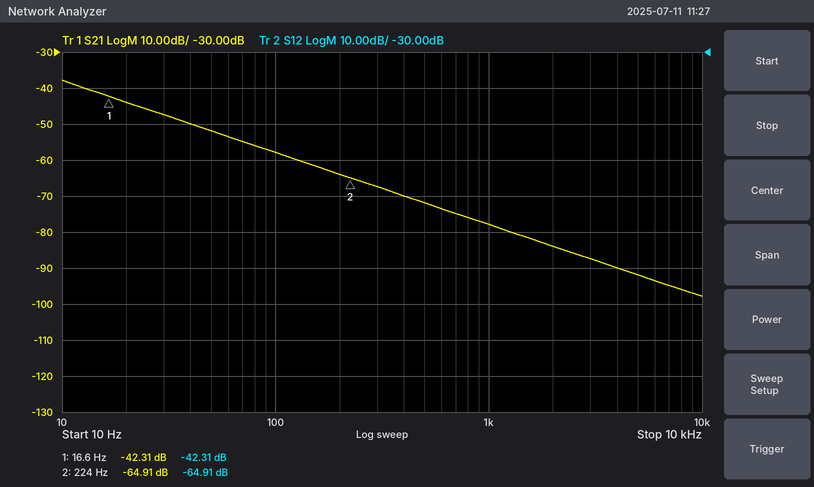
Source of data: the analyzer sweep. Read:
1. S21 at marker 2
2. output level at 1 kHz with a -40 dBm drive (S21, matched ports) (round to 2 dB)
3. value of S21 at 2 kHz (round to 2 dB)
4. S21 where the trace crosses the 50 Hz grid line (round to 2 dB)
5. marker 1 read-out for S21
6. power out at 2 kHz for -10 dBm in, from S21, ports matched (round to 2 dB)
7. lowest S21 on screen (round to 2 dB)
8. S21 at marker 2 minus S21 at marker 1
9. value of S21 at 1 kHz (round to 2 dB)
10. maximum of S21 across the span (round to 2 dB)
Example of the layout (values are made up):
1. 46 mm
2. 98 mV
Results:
1. -64.91 dB
2. -118 dBm
3. -84 dB
4. -52 dB
5. -42.31 dB
6. -94 dBm
7. -98 dB
8. -22.60 dB
9. -78 dB
10. -38 dB
